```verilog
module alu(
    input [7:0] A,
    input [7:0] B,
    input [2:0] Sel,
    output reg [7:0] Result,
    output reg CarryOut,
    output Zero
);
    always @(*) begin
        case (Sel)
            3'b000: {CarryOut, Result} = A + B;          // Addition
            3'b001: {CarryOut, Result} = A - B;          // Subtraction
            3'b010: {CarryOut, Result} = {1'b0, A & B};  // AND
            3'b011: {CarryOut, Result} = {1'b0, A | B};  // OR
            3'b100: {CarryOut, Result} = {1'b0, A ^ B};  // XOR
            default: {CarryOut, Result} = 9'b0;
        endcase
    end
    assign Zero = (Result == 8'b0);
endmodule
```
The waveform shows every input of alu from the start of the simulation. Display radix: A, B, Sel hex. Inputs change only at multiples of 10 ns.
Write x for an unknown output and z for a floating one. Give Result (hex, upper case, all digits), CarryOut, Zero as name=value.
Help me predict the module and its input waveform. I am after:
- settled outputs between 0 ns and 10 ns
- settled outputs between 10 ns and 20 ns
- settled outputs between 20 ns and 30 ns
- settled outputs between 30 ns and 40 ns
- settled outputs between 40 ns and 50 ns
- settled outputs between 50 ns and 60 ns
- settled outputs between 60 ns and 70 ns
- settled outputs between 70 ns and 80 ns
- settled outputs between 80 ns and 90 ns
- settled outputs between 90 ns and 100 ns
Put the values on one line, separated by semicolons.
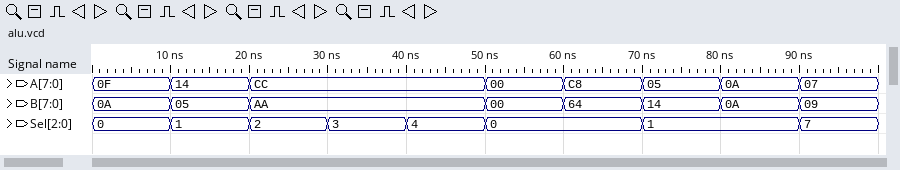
Result=19, CarryOut=0, Zero=0; Result=0F, CarryOut=0, Zero=0; Result=88, CarryOut=0, Zero=0; Result=EE, CarryOut=0, Zero=0; Result=66, CarryOut=0, Zero=0; Result=00, CarryOut=0, Zero=1; Result=2C, CarryOut=1, Zero=0; Result=F1, CarryOut=1, Zero=0; Result=00, CarryOut=0, Zero=1; Result=00, CarryOut=0, Zero=1
